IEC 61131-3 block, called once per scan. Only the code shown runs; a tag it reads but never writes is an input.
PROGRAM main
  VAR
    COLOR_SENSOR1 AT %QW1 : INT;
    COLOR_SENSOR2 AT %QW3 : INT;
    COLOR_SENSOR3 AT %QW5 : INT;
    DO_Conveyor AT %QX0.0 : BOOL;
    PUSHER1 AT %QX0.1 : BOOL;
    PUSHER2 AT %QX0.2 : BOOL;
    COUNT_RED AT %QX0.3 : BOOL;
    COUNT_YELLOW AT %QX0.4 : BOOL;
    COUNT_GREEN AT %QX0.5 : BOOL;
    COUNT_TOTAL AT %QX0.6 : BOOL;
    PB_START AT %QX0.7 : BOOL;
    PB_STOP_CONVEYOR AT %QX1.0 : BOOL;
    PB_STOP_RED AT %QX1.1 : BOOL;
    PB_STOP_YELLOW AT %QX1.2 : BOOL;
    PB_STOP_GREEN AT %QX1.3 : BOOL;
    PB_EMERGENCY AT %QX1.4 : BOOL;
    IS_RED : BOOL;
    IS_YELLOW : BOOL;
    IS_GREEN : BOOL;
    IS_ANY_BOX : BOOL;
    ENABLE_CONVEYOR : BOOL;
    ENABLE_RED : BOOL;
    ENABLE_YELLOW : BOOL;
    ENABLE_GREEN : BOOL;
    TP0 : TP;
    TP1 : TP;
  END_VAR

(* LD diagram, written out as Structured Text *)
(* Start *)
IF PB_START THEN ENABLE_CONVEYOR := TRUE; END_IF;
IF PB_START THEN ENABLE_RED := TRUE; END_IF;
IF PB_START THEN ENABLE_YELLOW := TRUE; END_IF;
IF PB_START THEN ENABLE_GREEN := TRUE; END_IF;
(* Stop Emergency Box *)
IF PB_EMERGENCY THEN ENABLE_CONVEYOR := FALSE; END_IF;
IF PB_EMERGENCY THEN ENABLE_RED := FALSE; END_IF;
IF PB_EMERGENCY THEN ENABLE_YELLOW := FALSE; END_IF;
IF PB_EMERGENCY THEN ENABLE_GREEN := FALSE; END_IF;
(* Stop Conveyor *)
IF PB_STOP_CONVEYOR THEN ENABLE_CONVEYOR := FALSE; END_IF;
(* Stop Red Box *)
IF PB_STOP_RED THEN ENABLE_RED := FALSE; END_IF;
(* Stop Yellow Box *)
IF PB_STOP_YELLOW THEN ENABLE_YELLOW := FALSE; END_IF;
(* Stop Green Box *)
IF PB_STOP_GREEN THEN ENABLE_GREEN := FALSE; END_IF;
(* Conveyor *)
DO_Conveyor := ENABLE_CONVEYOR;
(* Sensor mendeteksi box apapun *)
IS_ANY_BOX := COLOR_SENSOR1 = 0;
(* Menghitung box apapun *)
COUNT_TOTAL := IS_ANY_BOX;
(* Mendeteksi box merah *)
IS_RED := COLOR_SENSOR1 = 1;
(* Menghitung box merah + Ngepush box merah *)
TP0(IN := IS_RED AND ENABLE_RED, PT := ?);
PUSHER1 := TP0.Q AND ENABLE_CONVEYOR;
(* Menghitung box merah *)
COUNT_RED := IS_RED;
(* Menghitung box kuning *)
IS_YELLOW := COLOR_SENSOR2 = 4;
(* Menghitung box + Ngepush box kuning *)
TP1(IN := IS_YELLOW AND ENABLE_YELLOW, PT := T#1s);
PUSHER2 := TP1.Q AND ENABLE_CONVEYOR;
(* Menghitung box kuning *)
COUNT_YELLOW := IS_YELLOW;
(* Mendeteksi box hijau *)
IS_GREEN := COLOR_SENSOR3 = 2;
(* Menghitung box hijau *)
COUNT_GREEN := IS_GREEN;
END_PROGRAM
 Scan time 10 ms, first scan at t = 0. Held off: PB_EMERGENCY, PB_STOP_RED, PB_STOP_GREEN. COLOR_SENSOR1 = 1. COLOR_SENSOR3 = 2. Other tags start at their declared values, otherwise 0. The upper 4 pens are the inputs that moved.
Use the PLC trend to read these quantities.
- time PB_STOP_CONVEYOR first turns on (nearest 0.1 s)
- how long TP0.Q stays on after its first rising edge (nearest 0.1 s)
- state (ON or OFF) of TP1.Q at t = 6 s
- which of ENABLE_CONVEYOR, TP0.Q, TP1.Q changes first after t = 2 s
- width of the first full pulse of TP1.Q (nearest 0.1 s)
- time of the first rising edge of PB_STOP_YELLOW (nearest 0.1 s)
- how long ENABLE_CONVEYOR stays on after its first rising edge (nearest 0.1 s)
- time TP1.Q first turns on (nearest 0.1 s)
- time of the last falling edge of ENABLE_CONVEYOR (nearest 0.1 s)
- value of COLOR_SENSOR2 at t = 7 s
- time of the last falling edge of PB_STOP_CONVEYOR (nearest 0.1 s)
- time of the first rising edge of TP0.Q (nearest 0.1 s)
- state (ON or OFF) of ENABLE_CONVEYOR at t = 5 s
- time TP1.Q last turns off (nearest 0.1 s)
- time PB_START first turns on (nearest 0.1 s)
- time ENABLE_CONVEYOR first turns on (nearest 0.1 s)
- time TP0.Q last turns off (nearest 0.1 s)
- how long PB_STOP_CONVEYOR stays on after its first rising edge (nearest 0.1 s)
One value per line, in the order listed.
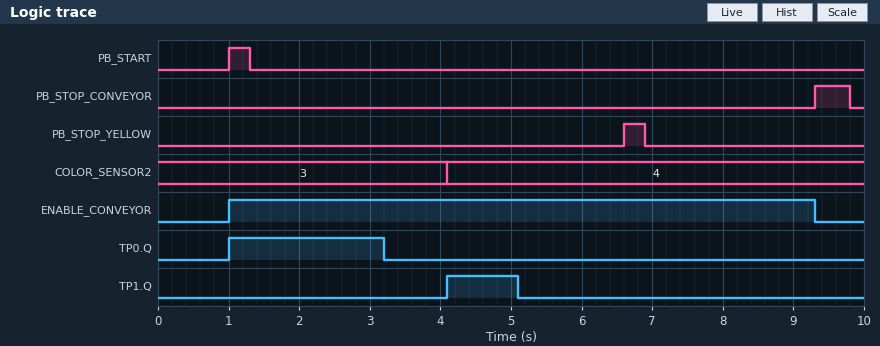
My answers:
9.3 s
2.2 s
OFF
TP0.Q
1.0 s
6.6 s
8.3 s
4.1 s
9.3 s
4
9.8 s
1.0 s
ON
5.1 s
1.0 s
1.0 s
3.2 s
0.5 s
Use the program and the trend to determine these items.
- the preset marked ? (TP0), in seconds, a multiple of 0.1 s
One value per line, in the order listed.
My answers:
2.2 s
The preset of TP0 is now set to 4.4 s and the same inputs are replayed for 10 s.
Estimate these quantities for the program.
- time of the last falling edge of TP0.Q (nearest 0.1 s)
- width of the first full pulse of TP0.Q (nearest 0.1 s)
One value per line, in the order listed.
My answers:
5.4 s
4.4 s
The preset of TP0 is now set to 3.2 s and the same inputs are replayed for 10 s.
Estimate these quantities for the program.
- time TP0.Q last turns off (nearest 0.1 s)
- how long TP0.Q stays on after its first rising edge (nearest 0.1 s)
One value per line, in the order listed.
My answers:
4.2 s
3.2 s
